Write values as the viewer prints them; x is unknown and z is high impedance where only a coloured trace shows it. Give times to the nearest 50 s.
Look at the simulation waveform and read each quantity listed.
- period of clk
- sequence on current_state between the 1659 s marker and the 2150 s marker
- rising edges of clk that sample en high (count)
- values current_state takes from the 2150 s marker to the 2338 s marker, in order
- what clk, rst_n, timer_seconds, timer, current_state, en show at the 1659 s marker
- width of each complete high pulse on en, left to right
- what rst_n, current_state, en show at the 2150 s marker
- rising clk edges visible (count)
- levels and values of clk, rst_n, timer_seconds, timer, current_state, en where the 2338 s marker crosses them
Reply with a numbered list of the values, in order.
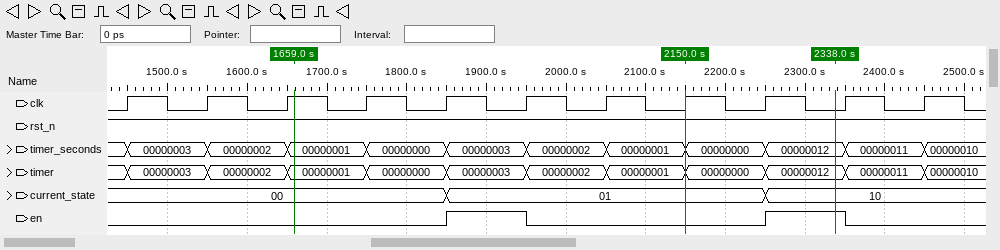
1. 100 s
2. 00, 01
3. 2
4. 01, 10
5. clk=1, rst_n=1, timer_seconds=00000001, timer=00000001, current_state=00, en=0
6. 100 s, 100 s
7. rst_n=1, current_state=01, en=0
8. 11
9. clk=0, rst_n=1, timer_seconds=00000012, timer=00000012, current_state=10, en=1
